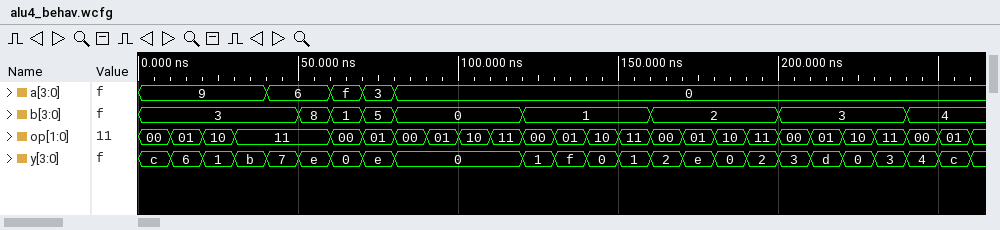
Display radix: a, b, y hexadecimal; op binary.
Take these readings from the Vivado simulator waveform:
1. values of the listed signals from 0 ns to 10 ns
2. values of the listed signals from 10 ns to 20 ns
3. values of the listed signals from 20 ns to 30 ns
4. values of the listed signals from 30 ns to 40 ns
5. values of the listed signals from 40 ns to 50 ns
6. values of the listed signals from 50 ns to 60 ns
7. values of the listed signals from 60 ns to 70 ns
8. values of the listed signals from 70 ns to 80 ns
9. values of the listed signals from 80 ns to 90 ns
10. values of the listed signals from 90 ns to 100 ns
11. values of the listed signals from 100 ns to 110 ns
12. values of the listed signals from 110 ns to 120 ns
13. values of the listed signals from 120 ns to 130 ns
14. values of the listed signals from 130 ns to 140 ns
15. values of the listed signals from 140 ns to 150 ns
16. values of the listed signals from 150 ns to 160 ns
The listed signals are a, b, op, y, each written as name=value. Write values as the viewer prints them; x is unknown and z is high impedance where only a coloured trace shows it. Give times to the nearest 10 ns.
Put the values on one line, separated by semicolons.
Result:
a=9, b=3, op=00, y=c; a=9, b=3, op=01, y=6; a=9, b=3, op=10, y=1; a=9, b=3, op=11, y=b; a=6, b=3, op=11, y=7; a=6, b=8, op=11, y=e; a=f, b=1, op=00, y=0; a=3, b=5, op=01, y=e; a=0, b=0, op=00, y=0; a=0, b=0, op=01, y=0; a=0, b=0, op=10, y=0; a=0, b=0, op=11, y=0; a=0, b=1, op=00, y=1; a=0, b=1, op=01, y=f; a=0, b=1, op=10, y=0; a=0, b=1, op=11, y=1
